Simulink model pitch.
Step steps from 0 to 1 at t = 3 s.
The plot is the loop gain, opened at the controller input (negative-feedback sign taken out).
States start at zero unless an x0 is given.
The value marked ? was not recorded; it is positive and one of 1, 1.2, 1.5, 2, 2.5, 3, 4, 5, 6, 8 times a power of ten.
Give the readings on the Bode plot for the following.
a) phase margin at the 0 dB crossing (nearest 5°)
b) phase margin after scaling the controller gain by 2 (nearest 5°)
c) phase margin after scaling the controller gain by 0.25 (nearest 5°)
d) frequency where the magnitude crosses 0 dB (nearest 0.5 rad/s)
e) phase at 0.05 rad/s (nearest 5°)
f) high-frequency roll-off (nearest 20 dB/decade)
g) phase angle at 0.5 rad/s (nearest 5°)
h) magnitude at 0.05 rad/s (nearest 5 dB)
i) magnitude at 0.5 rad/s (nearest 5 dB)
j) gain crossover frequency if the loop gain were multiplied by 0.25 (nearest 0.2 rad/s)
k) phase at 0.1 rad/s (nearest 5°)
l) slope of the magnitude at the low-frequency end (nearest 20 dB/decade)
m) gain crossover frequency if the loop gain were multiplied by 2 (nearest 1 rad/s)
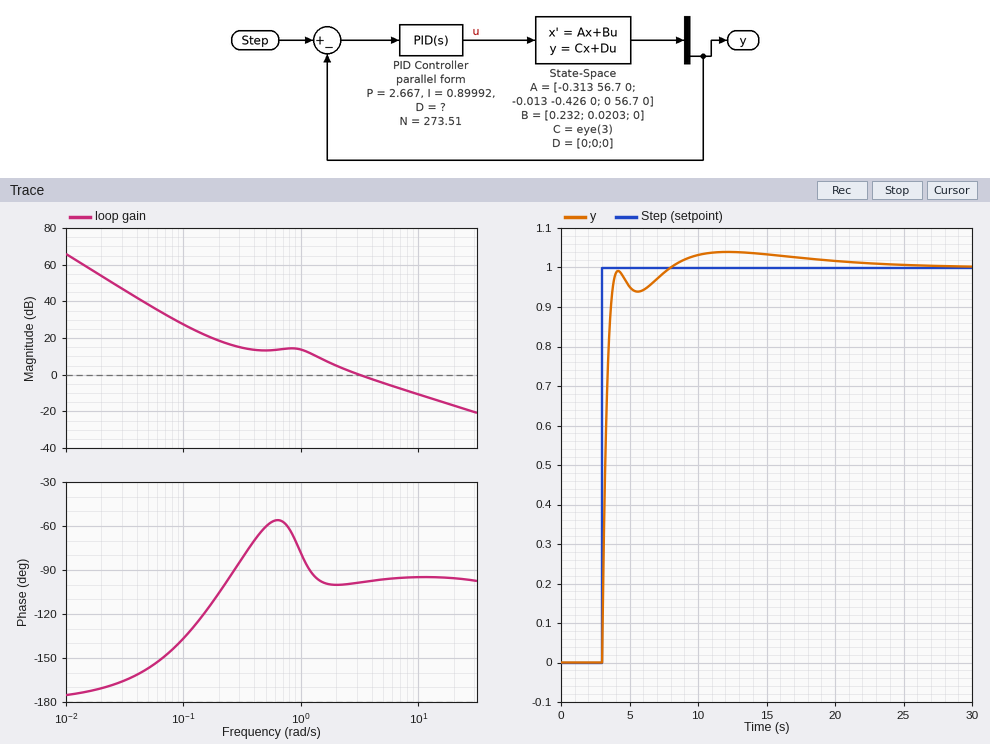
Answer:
80°
85°
90°
3.0 rad/s
-155°
-20 dB/decade
-60°
40 dB
15 dB
1.2 rad/s
-135°
-40 dB/decade
6 rad/s
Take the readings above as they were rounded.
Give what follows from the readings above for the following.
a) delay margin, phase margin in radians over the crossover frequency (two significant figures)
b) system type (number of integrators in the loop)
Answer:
0.47 s
2
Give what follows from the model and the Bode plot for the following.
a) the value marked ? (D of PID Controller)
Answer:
2.5
